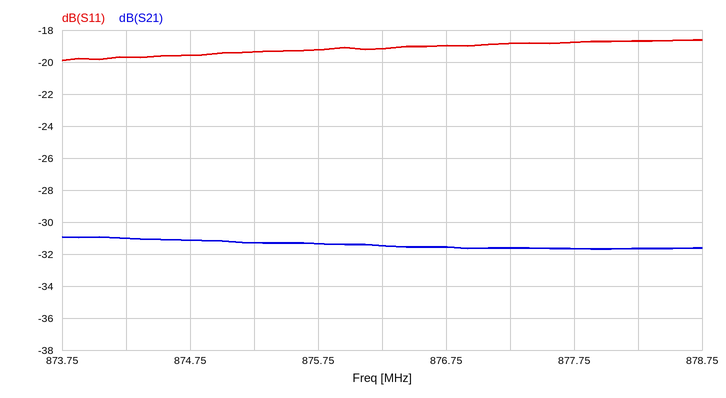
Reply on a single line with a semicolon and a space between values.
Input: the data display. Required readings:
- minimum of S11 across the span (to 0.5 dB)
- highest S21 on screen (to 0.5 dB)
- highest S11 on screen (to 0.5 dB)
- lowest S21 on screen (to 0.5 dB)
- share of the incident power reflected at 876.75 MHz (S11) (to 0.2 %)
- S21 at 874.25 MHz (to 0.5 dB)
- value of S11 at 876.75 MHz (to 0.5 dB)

-20.0 dB; -31.0 dB; -18.5 dB; -31.5 dB; 1.2 %; -31.0 dB; -19.0 dB
